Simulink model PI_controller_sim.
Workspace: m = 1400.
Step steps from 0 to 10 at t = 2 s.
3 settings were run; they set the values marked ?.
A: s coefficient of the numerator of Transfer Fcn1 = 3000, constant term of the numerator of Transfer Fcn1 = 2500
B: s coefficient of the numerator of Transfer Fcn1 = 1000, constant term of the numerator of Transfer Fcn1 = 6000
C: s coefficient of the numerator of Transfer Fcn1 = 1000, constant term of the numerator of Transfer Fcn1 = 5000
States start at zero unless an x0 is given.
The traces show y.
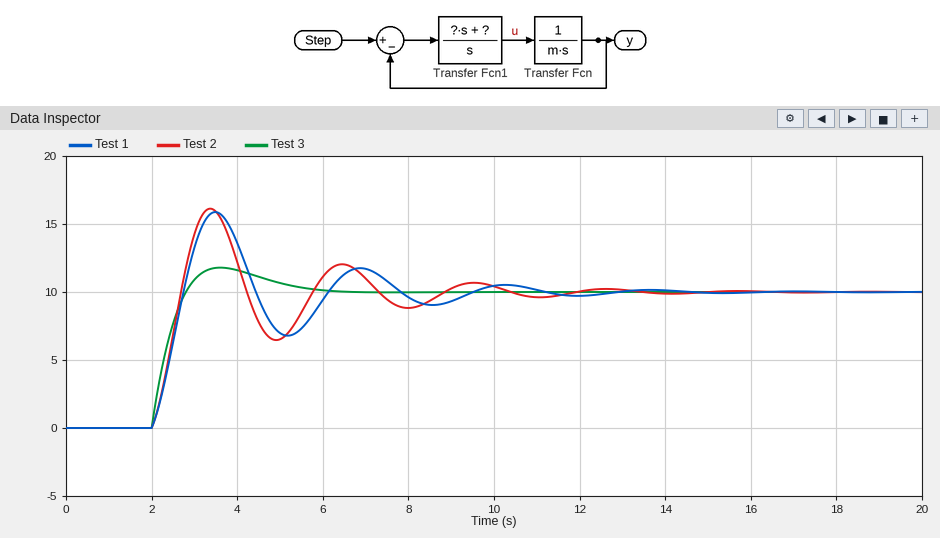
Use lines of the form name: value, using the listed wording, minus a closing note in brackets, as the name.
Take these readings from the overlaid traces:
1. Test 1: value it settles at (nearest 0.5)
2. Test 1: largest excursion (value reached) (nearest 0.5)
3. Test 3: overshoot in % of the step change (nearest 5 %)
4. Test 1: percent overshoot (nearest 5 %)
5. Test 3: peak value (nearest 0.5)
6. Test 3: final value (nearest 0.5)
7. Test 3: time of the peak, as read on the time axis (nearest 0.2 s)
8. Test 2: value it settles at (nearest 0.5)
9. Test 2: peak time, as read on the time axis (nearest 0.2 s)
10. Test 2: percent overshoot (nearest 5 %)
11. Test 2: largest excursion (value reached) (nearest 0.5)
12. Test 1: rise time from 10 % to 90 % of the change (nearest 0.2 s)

Test 1: value it settles at: 10.0
Test 1: largest excursion (value reached): 16.0
Test 3: overshoot in % of the step change: 20 %
Test 1: percent overshoot: 60 %
Test 3: peak value: 12.0
Test 3: final value: 10.0
Test 3: time of the peak, as read on the time axis: 3.6 s
Test 2: value it settles at: 10.0
Test 2: peak time, as read on the time axis: 3.4 s
Test 2: percent overshoot: 60 %
Test 2: largest excursion (value reached): 16.0
Test 1: rise time from 10 % to 90 % of the change: 0.6 s
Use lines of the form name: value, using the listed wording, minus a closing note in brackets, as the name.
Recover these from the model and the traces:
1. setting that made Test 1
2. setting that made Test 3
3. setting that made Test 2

setting that made Test 1: C
setting that made Test 3: A
setting that made Test 2: B
